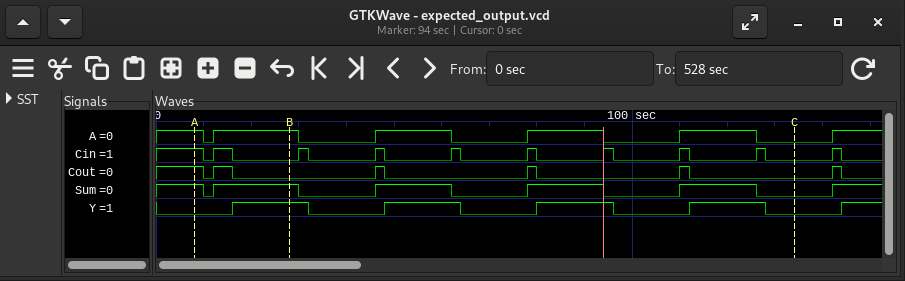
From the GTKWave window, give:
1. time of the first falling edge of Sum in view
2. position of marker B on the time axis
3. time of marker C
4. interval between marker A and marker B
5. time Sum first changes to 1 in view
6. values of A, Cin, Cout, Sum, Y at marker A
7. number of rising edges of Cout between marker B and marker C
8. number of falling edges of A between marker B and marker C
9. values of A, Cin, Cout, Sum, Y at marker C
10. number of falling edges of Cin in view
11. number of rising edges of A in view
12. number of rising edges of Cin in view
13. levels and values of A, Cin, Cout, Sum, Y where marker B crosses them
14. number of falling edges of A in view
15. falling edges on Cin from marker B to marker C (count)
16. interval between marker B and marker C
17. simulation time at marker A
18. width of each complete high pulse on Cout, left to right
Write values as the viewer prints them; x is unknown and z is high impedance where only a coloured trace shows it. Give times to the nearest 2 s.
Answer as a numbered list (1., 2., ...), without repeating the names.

1. 10 s
2. 28 s
3. 134 s
4. 20 s
5. 12 s
6. A=1, Cin=1, Cout=1, Sum=1, Y=0
7. 3
8. 4
9. A=0, Cin=0, Cout=0, Sum=0, Y=0
10. 10
11. 5
12. 9
13. A=1, Cin=0, Cout=0, Sum=1, Y=1
14. 5
15. 7
16. 106 s
17. 8 s
18. 4 s, 2 s, 2 s, 2 s, 2 s
